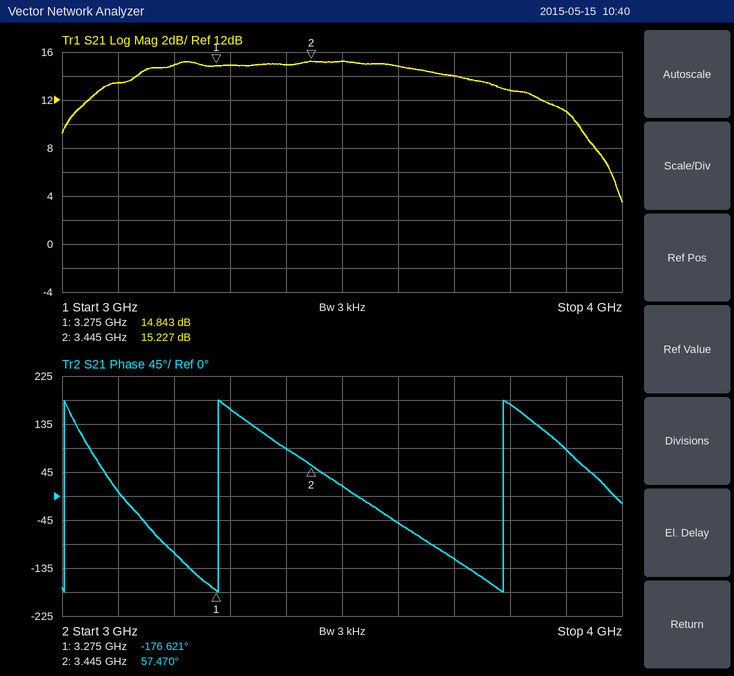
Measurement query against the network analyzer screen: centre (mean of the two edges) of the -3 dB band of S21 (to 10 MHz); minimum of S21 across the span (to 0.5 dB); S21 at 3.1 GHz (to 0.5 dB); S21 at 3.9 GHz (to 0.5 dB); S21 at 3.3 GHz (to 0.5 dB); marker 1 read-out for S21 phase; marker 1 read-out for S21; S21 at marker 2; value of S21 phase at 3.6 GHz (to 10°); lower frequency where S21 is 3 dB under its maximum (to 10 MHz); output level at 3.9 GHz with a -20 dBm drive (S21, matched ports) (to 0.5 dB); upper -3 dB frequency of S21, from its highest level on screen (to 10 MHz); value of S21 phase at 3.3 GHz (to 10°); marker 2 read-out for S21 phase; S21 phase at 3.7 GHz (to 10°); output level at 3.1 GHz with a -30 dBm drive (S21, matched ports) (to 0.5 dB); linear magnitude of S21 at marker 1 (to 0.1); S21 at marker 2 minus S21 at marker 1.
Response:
3.45 GHz
3.5 dB
13.5 dB
11.0 dB
15.0 dB
-176.621°
14.843 dB
15.227 dB
-50°
3.05 GHz
-9.0 dBm
3.85 GHz
160°
57.470°
-120°
-16.5 dBm
5.5
0.384 dB
